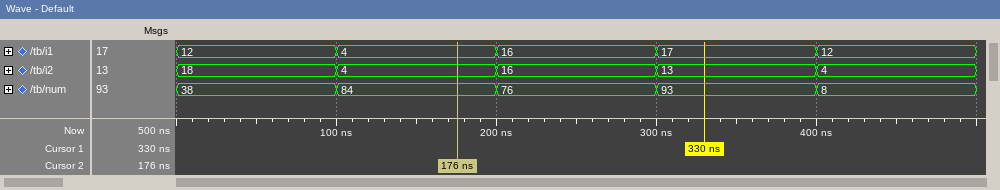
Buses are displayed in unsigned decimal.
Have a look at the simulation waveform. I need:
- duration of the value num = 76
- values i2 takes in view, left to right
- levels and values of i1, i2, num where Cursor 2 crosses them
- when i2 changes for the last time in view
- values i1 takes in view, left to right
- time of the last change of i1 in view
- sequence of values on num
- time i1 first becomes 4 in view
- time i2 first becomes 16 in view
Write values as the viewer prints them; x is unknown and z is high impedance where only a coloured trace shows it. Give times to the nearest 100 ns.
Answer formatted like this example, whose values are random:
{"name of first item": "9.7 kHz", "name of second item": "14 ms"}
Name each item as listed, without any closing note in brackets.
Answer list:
{"duration of the value num = 76": "100 ns", "values i2 takes in view, left to right": "18, 4, 16, 13, 4", "levels and values of i1, i2, num where Cursor 2 crosses them": "i1=4, i2=4, num=84", "when i2 changes for the last time in view": "400 ns", "values i1 takes in view, left to right": "12, 4, 16, 17, 12", "time of the last change of i1 in view": "400 ns", "sequence of values on num": "38, 84, 76, 93, 8", "time i1 first becomes 4 in view": "100 ns", "time i2 first becomes 16 in view": "200 ns"}
